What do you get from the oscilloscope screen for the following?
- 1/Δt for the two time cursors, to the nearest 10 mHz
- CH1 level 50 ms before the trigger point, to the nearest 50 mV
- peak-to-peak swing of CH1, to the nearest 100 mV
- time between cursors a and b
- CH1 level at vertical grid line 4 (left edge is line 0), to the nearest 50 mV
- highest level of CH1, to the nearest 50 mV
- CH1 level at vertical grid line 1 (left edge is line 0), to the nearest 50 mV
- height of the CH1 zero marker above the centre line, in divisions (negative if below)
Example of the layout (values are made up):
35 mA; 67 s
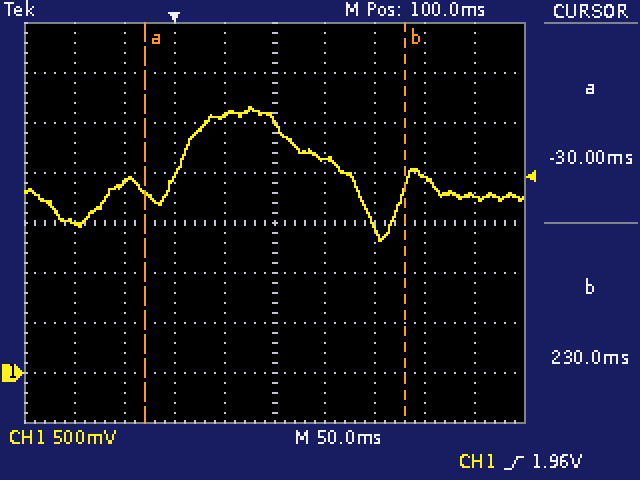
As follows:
3.85 Hz; 1.90 V; 1.30 V; 260 ms; 2.55 V; 2.65 V; 1.50 V; -3.0 div
